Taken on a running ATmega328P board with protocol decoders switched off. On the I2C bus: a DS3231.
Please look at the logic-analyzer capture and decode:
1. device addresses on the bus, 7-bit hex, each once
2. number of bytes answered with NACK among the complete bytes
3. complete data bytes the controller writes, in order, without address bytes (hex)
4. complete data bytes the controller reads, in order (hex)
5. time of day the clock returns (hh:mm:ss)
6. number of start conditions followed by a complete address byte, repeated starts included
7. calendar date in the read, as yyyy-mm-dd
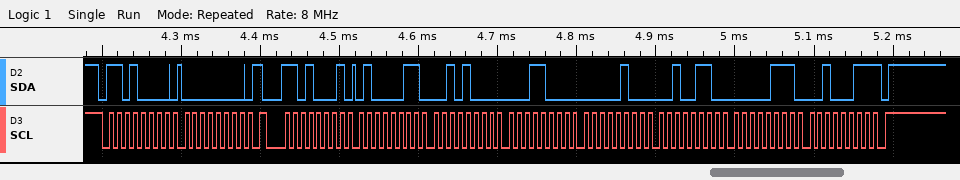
0x68
1
00
43 28 18 04 26 07 23
18:28:43
2
2023-07-26
